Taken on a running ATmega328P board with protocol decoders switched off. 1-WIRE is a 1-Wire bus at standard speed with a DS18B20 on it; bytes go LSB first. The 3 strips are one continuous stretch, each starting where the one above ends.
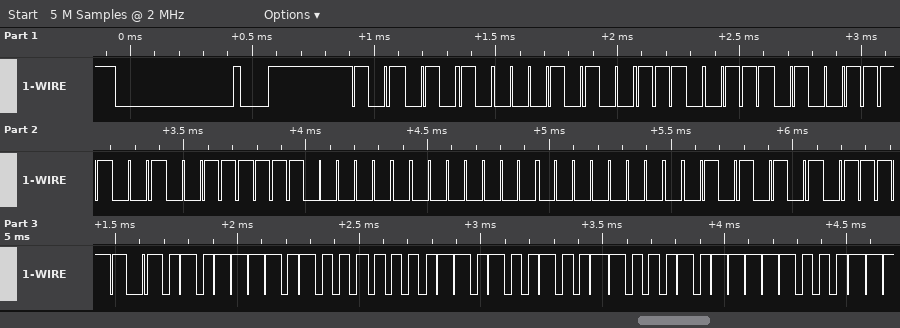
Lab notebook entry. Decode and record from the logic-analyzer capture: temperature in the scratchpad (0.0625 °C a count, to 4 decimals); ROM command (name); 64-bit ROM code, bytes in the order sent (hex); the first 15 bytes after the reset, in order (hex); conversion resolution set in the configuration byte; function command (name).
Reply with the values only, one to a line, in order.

23.6250 °C
Match ROM
28 E7 F2 E4 07 00 00 AA
55 28 E7 F2 E4 07 00 00 AA BE 7A 01 4B 46 1F
9 bits
Read Scratchpad
